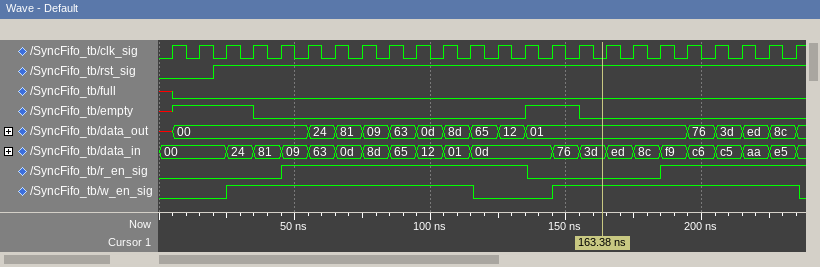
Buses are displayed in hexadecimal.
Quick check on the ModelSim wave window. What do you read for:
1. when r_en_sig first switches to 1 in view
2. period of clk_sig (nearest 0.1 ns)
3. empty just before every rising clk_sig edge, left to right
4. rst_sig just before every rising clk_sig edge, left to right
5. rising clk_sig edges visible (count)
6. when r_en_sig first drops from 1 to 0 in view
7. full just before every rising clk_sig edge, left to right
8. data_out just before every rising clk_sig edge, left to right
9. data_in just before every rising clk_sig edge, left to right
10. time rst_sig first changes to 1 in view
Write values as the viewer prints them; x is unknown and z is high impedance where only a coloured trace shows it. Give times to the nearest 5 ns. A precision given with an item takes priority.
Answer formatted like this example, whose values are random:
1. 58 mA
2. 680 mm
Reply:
1. 45 ns
2. 10 ns
3. x 1 1 1 0 0 0 0 0 0 0 0 0 0 1 1 0 0 0 0 0 0 0 0
4. 0 0 1 1 1 1 1 1 1 1 1 1 1 1 1 1 1 1 1 1 1 1 1 1
5. 24
6. 135 ns
7. x 0 0 0 0 0 0 0 0 0 0 0 0 0 0 0 0 0 0 0 0 0 0 0
8. x, 00, 00, 00, 00, 00, 24, 81, 09, 63, 0d, 8d, 65, 12, 01, 01, 01, 01, 01, 01, 76, 3d, ed, 8c
9. 00, 00, 00, 24, 81, 09, 63, 0d, 8d, 65, 12, 01, 0d, 0d, 0d, 76, 3d, ed, 8c, f9, c6, c5, aa, e5
10. 20 ns
